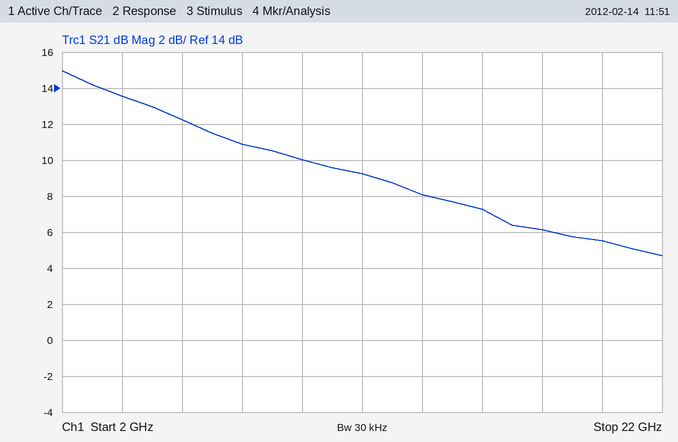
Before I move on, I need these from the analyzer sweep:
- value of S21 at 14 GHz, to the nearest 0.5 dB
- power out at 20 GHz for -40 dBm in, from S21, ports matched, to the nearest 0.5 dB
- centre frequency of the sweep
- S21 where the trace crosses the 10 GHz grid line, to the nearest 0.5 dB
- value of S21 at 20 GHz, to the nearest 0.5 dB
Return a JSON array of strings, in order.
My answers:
["8.0 dB", "-34.5 dBm", "12 GHz", "10.0 dB", "5.5 dB"]
